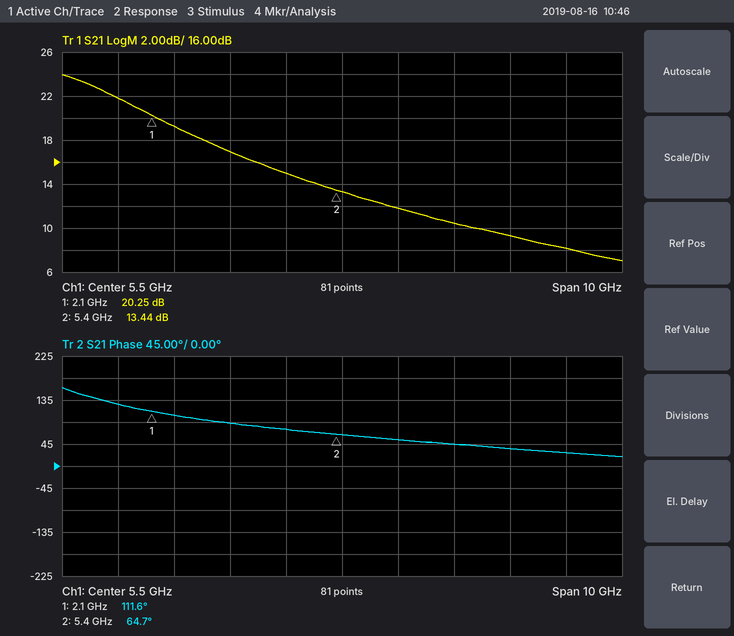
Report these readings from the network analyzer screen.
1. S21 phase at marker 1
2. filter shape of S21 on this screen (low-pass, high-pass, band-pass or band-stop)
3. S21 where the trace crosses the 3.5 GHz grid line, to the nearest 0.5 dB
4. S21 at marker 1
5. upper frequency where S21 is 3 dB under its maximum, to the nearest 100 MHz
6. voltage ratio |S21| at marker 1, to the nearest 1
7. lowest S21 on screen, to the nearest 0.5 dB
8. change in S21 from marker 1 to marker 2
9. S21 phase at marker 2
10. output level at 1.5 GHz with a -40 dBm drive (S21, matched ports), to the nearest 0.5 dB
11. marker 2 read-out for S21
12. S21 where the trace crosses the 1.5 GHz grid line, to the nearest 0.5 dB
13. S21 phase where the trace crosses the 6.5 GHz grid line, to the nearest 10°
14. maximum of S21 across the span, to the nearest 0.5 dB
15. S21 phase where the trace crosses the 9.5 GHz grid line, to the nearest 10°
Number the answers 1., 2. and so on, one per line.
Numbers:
1. 111.6°
2. low-pass
3. 17.0 dB
4. 20.25 dB
5. 1.8 GHz
6. 10
7. 7.0 dB
8. -6.81 dB
9. 64.7°
10. -18.0 dBm
11. 13.44 dB
12. 22.0 dB
13. 50°
14. 24.0 dB
15. 30°
